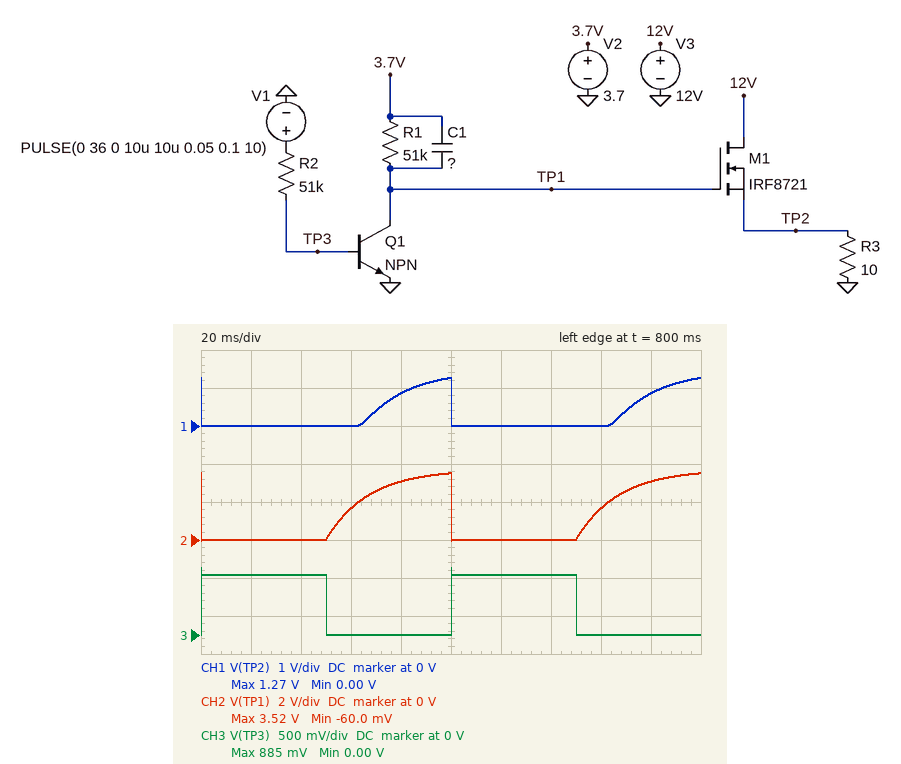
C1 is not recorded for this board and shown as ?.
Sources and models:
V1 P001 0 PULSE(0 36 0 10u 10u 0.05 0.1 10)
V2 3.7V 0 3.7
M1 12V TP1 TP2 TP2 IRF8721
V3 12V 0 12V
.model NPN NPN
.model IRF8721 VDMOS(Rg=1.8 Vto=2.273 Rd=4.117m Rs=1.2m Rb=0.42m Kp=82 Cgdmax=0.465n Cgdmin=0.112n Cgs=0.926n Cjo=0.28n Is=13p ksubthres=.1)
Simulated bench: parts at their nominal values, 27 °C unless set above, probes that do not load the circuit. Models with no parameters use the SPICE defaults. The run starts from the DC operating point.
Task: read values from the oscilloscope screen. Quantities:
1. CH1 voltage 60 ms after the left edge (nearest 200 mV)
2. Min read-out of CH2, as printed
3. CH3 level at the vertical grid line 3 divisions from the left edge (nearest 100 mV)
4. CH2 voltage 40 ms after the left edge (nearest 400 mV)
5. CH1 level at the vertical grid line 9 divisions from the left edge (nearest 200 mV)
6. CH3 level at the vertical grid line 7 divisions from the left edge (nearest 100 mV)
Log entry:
0 V
-60.0 mV
0 V
0 V
800 mV
800 mV
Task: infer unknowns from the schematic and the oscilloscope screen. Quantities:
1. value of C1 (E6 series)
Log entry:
330 nF
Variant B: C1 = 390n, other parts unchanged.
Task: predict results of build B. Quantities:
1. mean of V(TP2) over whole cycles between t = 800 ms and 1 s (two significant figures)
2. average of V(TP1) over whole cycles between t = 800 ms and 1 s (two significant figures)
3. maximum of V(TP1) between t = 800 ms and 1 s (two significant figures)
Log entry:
240 mV
1.2 V
3.4 V
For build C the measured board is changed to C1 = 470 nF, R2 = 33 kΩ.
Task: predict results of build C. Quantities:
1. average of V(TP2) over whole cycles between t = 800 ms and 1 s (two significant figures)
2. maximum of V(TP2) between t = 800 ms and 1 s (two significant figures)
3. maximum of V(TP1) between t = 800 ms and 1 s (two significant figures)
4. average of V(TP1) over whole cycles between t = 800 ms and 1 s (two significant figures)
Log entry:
180 mV
1.0 V
3.2 V
1.1 V
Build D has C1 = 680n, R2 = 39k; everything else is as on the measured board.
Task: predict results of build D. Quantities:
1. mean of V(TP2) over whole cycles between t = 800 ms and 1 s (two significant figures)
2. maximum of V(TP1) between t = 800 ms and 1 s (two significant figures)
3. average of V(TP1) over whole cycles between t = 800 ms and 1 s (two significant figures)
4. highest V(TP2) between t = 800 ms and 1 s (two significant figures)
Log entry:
74 mV
2.8 V
880 mV
630 mV
